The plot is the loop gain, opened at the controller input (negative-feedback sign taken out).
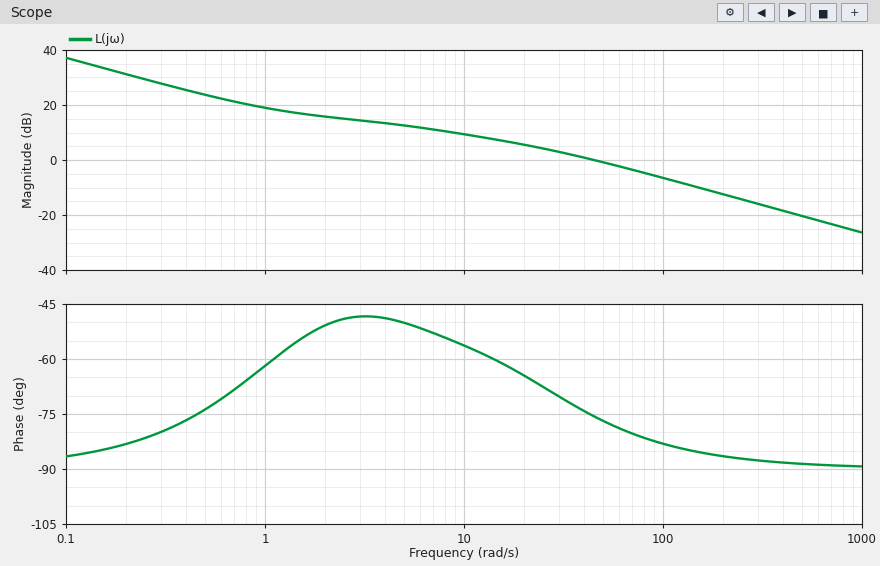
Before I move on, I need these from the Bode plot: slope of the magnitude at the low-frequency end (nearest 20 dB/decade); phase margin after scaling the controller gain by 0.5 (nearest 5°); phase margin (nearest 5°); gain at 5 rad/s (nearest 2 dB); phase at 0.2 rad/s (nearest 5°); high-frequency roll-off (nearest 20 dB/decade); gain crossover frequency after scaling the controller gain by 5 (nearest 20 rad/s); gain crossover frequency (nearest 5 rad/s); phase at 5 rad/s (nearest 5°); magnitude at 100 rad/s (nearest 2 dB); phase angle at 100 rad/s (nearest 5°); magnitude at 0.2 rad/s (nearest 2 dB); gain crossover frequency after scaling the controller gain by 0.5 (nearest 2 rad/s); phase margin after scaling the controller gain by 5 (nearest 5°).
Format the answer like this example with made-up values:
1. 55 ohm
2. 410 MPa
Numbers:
1. -20 dB/decade
2. 115°
3. 105°
4. 12 dB
5. -85°
6. -20 dB/decade
7. 240 rad/s
8. 45 rad/s
9. -50°
10. -6 dB
11. -85°
12. 32 dB
13. 18 rad/s
14. 95°
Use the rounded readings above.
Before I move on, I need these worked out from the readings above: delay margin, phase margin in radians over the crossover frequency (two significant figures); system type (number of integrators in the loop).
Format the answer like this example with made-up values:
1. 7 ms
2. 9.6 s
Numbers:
1. 0.041 s
2. 1
